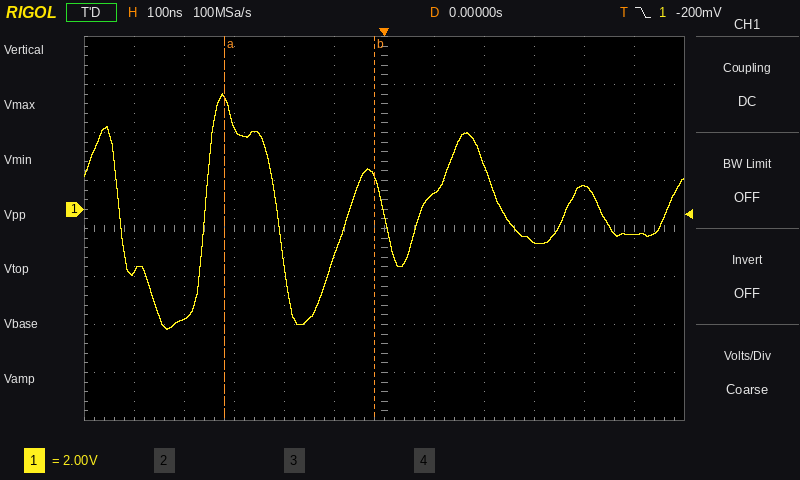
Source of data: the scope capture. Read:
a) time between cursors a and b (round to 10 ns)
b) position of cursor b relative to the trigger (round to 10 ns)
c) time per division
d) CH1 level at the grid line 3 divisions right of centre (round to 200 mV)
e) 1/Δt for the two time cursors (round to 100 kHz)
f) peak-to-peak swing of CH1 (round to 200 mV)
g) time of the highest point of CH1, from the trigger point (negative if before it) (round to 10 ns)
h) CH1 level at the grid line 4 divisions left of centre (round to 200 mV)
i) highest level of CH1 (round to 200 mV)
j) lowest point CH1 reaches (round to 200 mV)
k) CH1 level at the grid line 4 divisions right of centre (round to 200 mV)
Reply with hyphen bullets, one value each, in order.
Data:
- 300 ns
- -20 ns
- 100 ns
- -1.4 V
- 3.3 MHz
- 9.8 V
- -320 ns
- -4.6 V
- 4.8 V
- -5.0 V
- 1.0 V
